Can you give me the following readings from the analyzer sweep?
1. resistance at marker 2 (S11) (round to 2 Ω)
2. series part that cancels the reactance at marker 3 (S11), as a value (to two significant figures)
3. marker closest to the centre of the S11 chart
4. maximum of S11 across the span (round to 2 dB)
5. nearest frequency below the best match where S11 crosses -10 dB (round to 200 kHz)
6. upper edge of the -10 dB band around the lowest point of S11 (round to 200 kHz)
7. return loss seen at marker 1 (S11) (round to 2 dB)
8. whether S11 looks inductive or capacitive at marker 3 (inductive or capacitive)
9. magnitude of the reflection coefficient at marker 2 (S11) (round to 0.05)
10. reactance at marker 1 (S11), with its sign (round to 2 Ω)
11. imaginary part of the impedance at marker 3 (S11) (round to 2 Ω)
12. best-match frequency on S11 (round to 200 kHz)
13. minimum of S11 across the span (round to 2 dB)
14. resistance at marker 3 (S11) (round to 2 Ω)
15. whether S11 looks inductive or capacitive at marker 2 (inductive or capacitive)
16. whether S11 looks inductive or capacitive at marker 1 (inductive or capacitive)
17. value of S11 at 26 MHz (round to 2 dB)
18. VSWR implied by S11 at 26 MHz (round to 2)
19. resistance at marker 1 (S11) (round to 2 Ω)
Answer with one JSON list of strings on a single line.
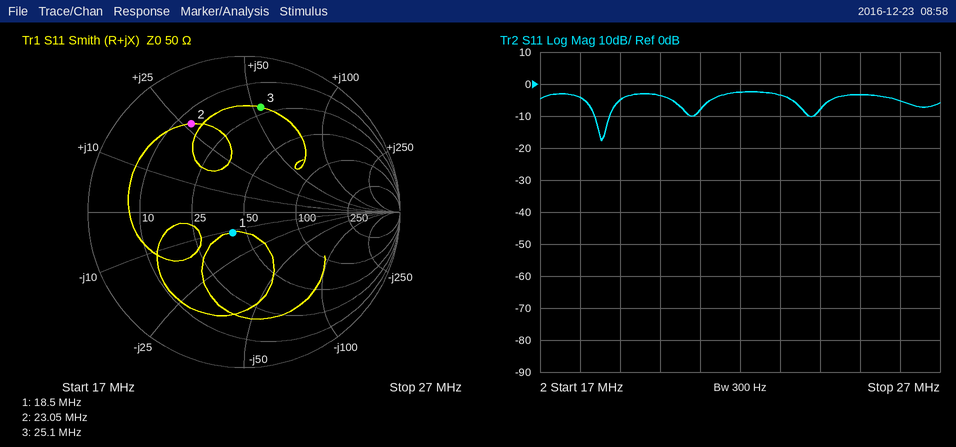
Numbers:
["14 Ω", "120 pF", "marker 1", "-2 dB", "18.4 MHz", "18.8 MHz", "16 dB", "inductive", "0.65", "-12 Ω", "+54 Ω", "18.6 MHz", "-18 dB", "22 Ω", "inductive", "capacitive", "-6 dB", "4", "42 Ω"]
